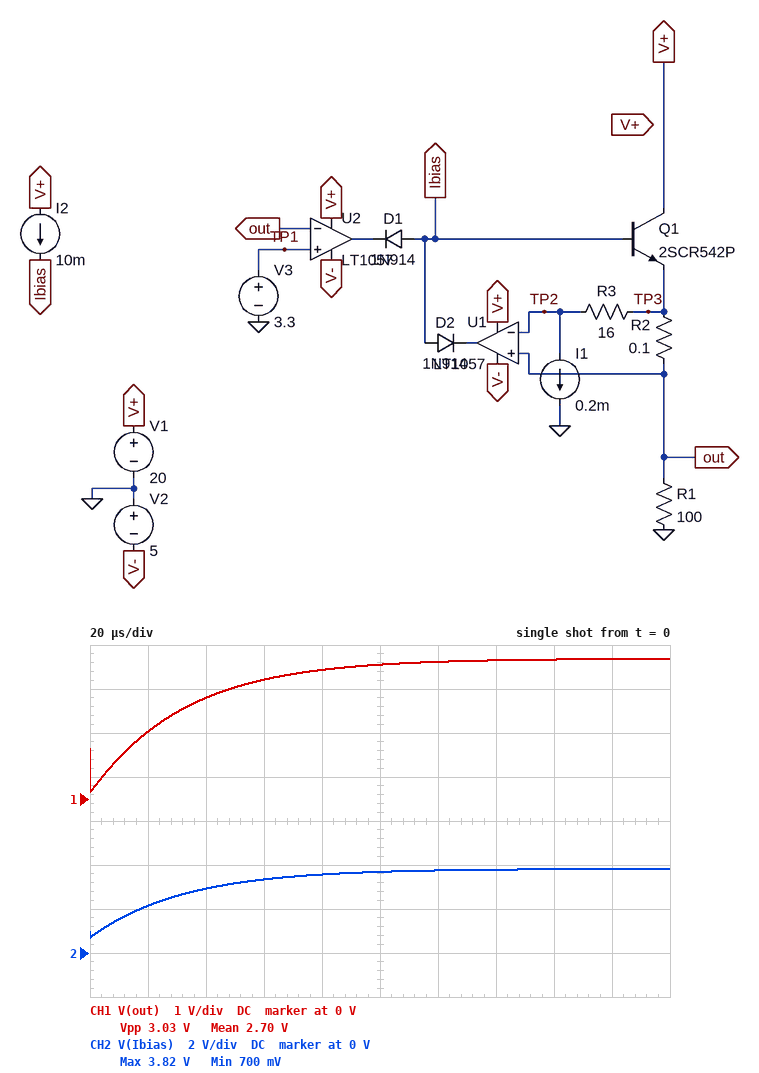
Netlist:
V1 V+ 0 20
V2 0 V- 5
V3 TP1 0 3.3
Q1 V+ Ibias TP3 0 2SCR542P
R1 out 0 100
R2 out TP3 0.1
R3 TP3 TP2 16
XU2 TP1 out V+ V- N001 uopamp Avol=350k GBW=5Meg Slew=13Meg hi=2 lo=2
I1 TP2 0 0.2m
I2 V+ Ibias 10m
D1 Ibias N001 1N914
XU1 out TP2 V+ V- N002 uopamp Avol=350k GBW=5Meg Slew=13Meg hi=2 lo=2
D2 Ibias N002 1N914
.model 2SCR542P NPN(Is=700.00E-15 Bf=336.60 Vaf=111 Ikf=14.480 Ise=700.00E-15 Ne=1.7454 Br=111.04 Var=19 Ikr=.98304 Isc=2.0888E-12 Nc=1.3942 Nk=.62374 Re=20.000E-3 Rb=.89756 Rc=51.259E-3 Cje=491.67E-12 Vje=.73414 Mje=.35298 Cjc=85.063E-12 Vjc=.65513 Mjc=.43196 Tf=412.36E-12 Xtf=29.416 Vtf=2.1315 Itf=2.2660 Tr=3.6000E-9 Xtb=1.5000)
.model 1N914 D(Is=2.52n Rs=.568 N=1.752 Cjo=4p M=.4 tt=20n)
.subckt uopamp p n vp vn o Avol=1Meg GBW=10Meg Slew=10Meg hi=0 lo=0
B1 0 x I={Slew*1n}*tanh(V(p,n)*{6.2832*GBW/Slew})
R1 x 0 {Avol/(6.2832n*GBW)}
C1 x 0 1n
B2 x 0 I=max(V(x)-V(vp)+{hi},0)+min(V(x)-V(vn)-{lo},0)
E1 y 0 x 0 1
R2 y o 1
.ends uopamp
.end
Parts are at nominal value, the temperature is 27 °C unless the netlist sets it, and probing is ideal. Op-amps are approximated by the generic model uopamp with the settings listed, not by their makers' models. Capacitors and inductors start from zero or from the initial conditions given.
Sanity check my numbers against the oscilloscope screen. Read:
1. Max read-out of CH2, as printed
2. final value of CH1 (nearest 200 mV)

3.82 V
3.2 V
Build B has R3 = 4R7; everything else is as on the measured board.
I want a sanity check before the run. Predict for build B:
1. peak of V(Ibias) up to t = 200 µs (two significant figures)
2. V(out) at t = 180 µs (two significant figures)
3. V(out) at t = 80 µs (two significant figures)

1.5 V
930 mV
870 mV
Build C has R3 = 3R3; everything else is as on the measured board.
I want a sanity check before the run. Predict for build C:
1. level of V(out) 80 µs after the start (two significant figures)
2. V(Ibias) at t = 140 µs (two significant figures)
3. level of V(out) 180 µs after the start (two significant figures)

610 mV
1.2 V
660 mV
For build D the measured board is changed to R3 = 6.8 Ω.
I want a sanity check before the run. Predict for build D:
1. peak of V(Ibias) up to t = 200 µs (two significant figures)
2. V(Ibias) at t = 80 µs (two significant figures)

2.0 V
1.9 V
